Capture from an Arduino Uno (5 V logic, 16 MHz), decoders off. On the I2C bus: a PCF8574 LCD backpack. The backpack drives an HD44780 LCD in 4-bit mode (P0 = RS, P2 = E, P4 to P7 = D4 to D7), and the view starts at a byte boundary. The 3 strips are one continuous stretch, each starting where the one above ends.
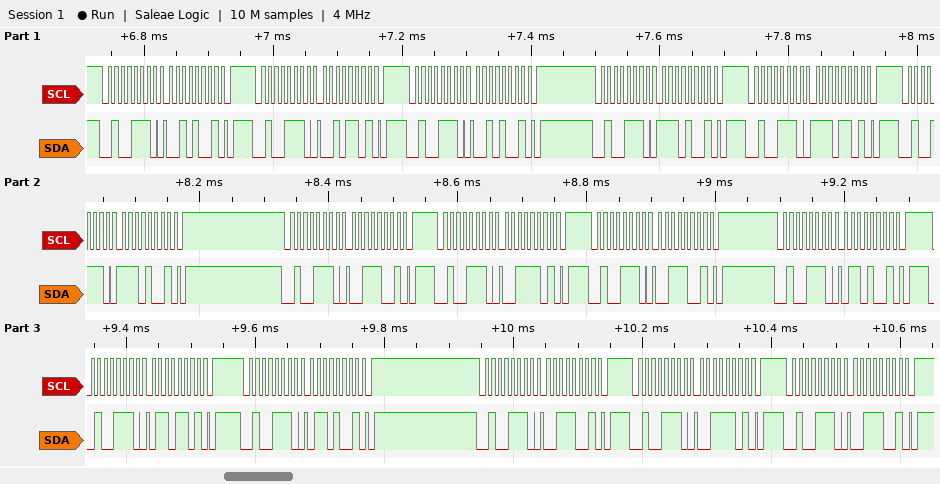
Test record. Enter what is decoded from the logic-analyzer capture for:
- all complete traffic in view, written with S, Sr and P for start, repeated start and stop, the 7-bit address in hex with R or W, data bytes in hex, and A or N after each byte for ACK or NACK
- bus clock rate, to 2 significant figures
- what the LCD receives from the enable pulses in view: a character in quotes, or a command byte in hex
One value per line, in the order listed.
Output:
S 27W A 29 A P S 27W A 2D A P S 27W A 29 A P S 27W A E9 A P S 27W A ED A P S 27W A E9 A P S 27W A 39 A P S 27W A 3D A P S 27W A 39 A P S 27W A 69 A P S 27W A 6D A P S 27W A 69 A P S 27W A 39 A P S 27W A 3D A P S 27W A 39 A P
100 kHz
'.' '6'
